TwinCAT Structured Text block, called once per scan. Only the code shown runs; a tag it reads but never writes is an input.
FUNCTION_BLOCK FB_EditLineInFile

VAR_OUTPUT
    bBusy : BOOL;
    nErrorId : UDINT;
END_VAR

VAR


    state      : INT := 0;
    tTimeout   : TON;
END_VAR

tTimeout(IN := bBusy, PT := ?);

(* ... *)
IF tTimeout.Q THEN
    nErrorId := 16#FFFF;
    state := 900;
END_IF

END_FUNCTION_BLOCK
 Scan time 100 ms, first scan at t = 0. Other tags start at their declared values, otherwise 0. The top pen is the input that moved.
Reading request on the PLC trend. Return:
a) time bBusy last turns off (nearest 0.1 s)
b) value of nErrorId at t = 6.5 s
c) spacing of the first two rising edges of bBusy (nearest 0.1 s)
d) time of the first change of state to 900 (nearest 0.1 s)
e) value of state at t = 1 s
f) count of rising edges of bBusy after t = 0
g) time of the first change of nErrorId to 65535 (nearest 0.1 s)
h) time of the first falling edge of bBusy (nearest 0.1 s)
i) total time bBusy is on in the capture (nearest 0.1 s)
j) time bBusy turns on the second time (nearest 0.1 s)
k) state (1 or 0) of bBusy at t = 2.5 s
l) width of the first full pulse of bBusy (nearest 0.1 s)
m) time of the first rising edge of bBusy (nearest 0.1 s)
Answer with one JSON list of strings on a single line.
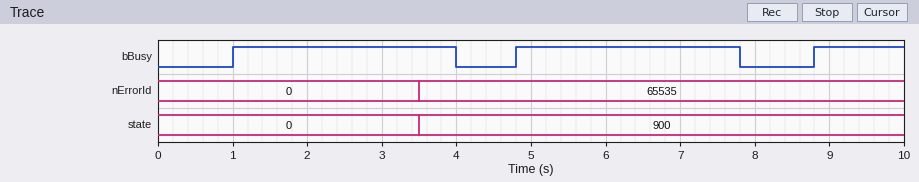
["7.8 s", "65535", "3.8 s", "3.5 s", "0", "3", "3.5 s", "4.0 s", "7.2 s", "4.8 s", "1", "3.0 s", "1.0 s"]
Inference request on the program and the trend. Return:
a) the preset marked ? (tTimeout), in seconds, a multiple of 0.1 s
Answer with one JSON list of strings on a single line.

["2.5 s"]
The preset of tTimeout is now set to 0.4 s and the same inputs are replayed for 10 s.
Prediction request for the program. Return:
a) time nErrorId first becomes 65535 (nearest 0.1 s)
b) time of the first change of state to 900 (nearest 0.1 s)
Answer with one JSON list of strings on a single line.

["1.4 s", "1.4 s"]
